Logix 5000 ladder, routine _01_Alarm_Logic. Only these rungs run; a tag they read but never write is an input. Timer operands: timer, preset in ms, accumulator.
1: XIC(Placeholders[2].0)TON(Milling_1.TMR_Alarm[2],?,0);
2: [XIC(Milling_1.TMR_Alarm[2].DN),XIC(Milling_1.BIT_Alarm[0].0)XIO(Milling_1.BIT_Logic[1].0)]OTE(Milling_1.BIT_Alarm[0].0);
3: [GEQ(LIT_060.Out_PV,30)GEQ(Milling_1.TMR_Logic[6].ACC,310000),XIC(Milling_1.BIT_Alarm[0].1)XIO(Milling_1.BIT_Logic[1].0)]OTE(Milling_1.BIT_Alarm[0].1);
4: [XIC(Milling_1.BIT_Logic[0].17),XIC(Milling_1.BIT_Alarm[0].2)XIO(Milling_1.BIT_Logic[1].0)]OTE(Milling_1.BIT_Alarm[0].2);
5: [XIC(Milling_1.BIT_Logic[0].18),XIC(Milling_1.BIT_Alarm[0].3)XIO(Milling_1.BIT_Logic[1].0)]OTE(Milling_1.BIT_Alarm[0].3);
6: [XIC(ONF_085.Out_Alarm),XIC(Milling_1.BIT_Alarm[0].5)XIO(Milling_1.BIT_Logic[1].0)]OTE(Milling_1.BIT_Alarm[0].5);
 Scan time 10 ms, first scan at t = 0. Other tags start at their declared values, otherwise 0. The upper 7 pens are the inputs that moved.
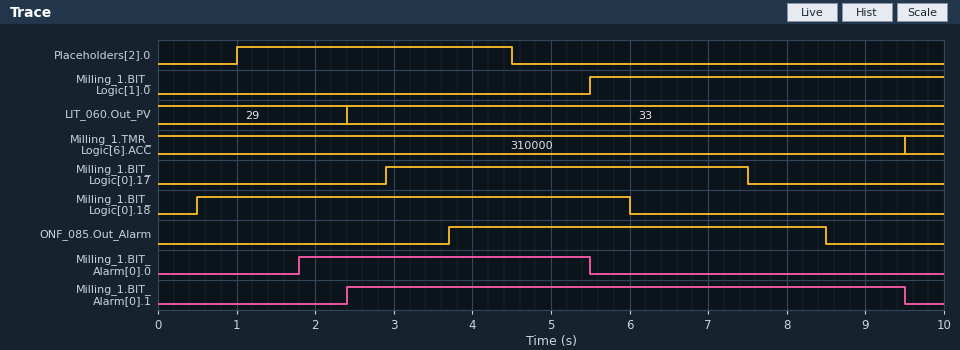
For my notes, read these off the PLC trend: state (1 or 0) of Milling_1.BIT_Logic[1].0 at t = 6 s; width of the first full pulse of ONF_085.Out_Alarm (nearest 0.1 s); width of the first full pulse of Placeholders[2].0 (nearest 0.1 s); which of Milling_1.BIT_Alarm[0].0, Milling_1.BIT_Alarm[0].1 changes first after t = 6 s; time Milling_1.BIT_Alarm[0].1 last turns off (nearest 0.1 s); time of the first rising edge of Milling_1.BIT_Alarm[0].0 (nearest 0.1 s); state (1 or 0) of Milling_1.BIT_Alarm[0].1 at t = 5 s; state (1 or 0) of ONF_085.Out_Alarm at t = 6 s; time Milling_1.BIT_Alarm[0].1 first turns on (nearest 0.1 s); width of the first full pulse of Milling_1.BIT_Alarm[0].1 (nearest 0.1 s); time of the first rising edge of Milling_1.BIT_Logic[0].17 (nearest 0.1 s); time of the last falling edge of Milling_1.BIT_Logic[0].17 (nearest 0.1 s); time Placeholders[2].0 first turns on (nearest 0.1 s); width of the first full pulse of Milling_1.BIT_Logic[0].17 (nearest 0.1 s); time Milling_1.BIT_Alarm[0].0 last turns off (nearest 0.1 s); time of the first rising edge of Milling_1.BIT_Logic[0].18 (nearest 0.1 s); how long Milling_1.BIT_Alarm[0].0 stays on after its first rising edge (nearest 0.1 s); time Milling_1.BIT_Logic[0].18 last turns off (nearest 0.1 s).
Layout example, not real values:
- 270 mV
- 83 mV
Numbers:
- 1
- 4.8 s
- 3.5 s
- Milling_1.BIT_Alarm[0].1
- 9.5 s
- 1.8 s
- 1
- 1
- 2.4 s
- 7.1 s
- 2.9 s
- 7.5 s
- 1.0 s
- 4.6 s
- 5.5 s
- 0.5 s
- 3.7 s
- 6.0 s
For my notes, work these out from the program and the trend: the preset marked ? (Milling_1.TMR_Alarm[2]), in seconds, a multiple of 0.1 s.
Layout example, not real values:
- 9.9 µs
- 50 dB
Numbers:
- 0.8 s
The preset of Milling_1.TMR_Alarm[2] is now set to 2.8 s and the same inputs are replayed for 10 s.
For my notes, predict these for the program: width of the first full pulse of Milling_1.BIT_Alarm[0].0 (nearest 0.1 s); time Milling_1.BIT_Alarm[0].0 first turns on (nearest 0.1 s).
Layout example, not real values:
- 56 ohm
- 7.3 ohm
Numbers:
- 1.7 s
- 3.8 s
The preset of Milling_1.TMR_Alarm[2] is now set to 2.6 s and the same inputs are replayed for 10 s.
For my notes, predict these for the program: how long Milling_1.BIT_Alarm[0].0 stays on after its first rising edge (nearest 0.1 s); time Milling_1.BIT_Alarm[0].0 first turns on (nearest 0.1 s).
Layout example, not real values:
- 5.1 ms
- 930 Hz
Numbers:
- 1.9 s
- 3.6 s
